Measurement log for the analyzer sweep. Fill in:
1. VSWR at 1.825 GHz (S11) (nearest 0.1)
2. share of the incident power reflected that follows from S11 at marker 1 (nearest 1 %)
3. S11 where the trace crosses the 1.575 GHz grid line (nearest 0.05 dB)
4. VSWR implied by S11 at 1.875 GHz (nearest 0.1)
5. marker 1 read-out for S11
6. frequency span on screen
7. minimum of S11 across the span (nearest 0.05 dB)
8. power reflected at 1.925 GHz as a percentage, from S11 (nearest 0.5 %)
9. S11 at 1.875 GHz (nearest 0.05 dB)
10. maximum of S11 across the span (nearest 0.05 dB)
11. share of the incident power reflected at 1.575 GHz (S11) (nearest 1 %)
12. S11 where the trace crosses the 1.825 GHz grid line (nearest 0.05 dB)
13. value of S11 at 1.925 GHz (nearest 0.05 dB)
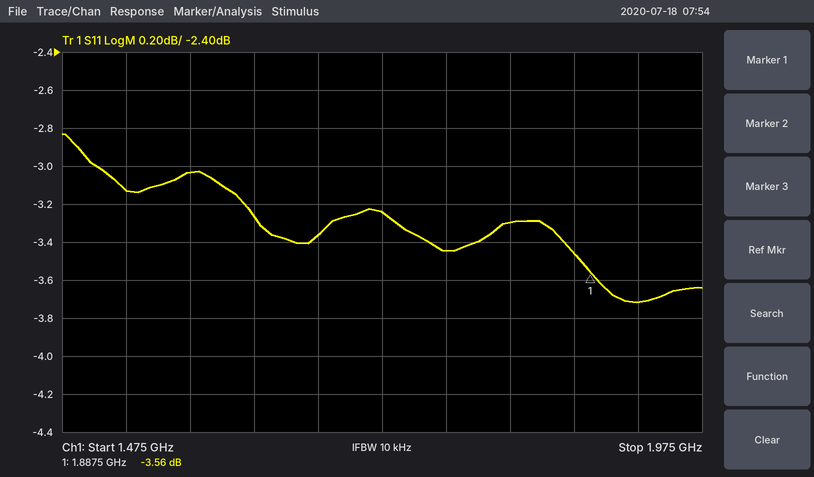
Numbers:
5.3
44 %
-3.05 dB
5.1
-3.56 dB
500 MHz
-3.70 dB
42.5 %
-3.45 dB
-2.85 dB
50 %
-3.30 dB
-3.70 dB
